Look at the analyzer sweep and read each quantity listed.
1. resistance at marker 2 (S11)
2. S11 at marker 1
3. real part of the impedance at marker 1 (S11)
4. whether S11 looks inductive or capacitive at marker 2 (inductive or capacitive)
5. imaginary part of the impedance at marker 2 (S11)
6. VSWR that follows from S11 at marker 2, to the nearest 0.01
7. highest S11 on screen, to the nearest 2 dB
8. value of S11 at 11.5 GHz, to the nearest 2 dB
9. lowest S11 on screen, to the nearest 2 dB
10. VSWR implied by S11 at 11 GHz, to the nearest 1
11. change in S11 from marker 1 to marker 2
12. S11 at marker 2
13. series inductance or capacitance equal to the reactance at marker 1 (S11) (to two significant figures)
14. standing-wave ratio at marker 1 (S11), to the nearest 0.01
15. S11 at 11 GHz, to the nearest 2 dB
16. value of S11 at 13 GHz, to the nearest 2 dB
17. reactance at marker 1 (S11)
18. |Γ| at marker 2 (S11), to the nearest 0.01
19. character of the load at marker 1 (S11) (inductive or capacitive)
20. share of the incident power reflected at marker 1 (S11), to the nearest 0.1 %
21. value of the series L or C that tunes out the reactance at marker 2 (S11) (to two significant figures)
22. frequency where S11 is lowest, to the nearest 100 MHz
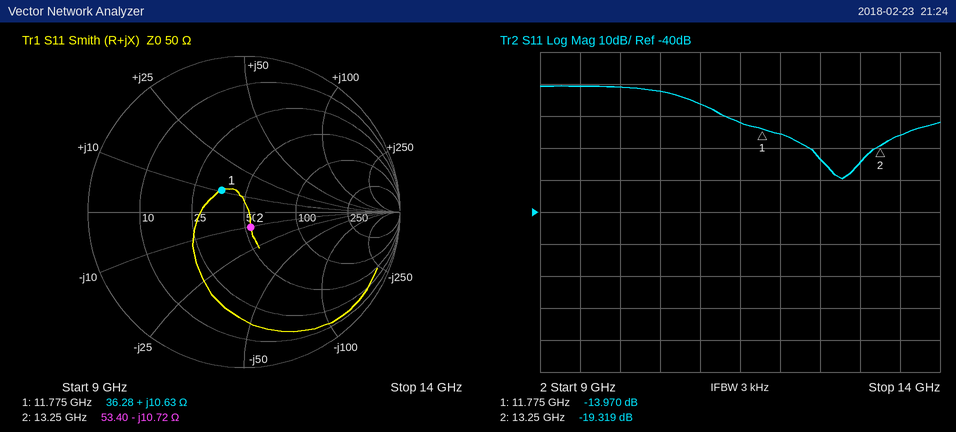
53.40 Ω
-13.970 dB
36.28 Ω
capacitive
-10.72 Ω
1.24
0 dB
-12 dB
-30 dB
3
-5.349 dB
-19.319 dB
140 pH
1.50
-6 dB
-24 dB
+10.63 Ω
0.11
inductive
4.0 %
130 pH
12.8 GHz
